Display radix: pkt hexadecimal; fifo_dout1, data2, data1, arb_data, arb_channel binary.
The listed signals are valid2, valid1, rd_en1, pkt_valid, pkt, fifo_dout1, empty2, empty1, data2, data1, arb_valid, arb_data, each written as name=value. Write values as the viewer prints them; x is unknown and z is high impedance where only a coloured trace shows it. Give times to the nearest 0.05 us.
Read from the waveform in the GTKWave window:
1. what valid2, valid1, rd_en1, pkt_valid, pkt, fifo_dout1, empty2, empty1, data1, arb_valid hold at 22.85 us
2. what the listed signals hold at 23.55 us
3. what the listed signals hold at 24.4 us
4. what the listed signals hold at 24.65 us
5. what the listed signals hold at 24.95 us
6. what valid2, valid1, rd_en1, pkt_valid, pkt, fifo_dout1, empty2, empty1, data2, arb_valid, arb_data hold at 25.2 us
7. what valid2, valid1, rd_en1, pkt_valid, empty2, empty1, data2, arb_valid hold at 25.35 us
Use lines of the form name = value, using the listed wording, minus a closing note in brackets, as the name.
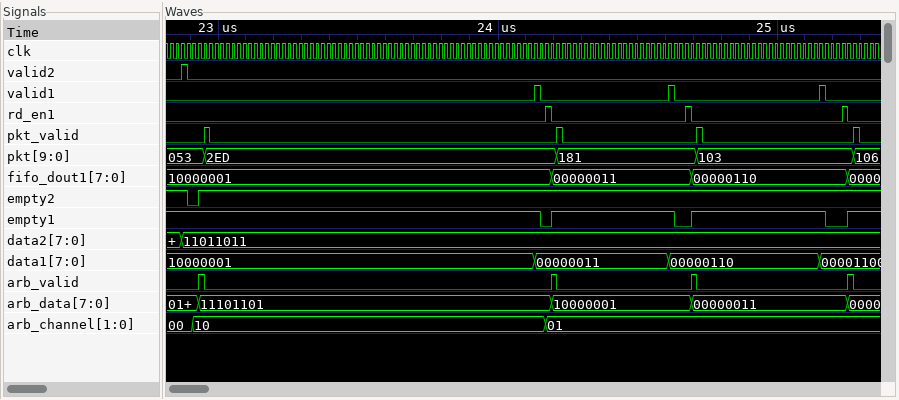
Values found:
what valid2, valid1, rd_en1, pkt_valid, pkt, fifo_dout1, empty2, empty1, data1, arb_valid hold at 22.85 us = valid2=0, valid1=0, rd_en1=0, pkt_valid=0, pkt=053, fifo_dout1=10000001, empty2=1, empty1=1, data1=10000001, arb_valid=0
what the listed signals hold at 23.55 us = valid2=0, valid1=0, rd_en1=0, pkt_valid=0, pkt=2ED, fifo_dout1=10000001, empty2=1, empty1=1, data2=11011011, data1=10000001, arb_valid=0, arb_data=11101101
what the listed signals hold at 24.4 us = valid2=0, valid1=0, rd_en1=0, pkt_valid=0, pkt=181, fifo_dout1=00000011, empty2=1, empty1=1, data2=11011011, data1=00000011, arb_valid=0, arb_data=10000001
what the listed signals hold at 24.65 us = valid2=0, valid1=0, rd_en1=0, pkt_valid=0, pkt=181, fifo_dout1=00000011, empty2=1, empty1=0, data2=11011011, data1=00000110, arb_valid=0, arb_data=10000001
what the listed signals hold at 24.95 us = valid2=0, valid1=0, rd_en1=0, pkt_valid=0, pkt=103, fifo_dout1=00000110, empty2=1, empty1=1, data2=11011011, data1=00000110, arb_valid=0, arb_data=00000011
what valid2, valid1, rd_en1, pkt_valid, pkt, fifo_dout1, empty2, empty1, data2, arb_valid, arb_data hold at 25.2 us = valid2=0, valid1=0, rd_en1=0, pkt_valid=0, pkt=103, fifo_dout1=00000110, empty2=1, empty1=0, data2=11011011, arb_valid=0, arb_data=00000011
what valid2, valid1, rd_en1, pkt_valid, empty2, empty1, data2, arb_valid hold at 25.35 us = valid2=0, valid1=0, rd_en1=0, pkt_valid=0, empty2=1, empty1=1, data2=11011011, arb_valid=0
